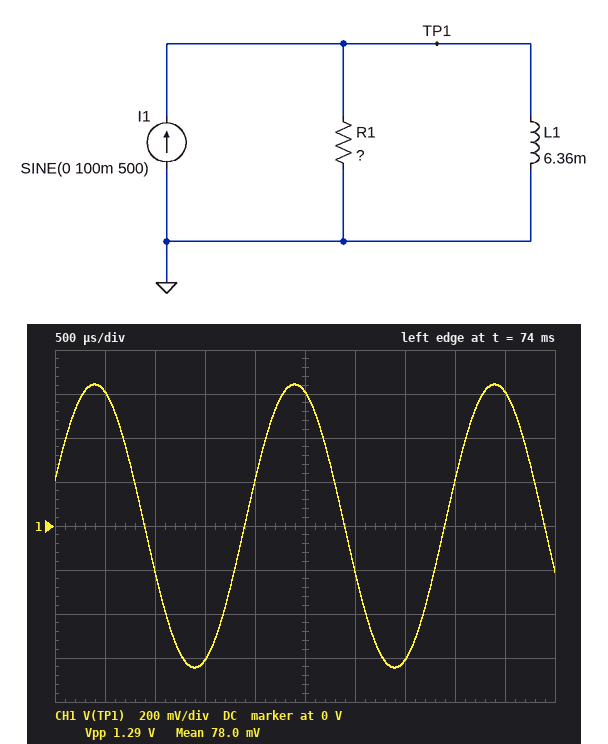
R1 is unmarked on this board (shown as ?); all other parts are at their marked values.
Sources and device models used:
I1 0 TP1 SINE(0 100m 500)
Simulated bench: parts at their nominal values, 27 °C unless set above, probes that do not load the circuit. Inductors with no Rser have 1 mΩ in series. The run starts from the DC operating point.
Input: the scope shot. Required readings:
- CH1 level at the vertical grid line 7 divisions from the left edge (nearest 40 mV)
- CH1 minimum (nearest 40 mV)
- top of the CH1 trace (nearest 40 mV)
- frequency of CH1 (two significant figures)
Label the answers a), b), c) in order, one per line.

a) -600 mV
b) -640 mV
c) 640 mV
d) 500 Hz
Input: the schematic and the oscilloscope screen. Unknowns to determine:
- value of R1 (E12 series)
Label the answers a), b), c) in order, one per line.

a) 6.8 Ω
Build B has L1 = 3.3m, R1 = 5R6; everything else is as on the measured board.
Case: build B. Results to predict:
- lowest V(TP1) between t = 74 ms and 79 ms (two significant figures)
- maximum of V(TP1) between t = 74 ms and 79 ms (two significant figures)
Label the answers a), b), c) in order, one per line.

a) -490 mV
b) 490 mV
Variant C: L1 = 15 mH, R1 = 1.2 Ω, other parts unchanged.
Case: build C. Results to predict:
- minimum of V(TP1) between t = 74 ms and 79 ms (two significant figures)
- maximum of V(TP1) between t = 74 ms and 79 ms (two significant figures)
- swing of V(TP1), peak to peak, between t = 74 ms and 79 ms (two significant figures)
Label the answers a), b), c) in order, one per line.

a) -120 mV
b) 120 mV
c) 240 mV
